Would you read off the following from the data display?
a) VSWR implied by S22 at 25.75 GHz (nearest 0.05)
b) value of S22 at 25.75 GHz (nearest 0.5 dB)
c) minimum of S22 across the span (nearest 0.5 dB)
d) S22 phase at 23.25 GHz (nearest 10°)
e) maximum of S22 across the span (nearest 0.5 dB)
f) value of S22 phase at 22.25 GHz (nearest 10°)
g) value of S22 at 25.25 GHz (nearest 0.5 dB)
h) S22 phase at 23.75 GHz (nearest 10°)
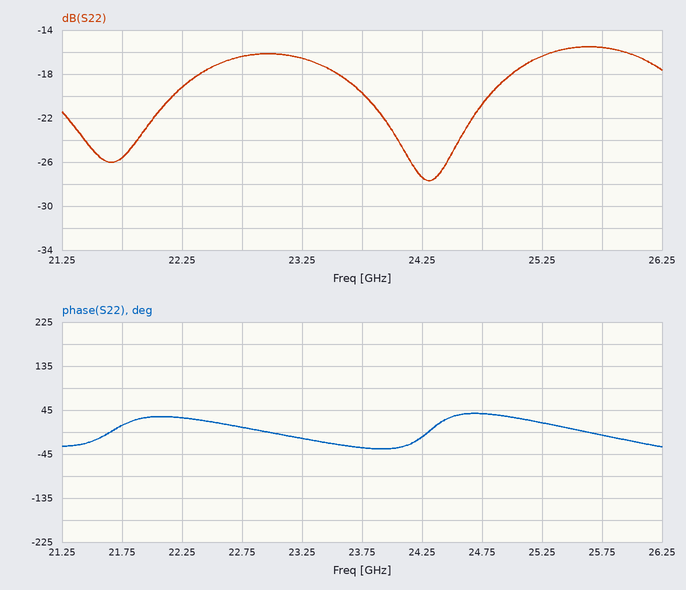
1.40
-15.5 dB
-27.5 dB
-10°
-15.5 dB
30°
-16.5 dB
-30°
